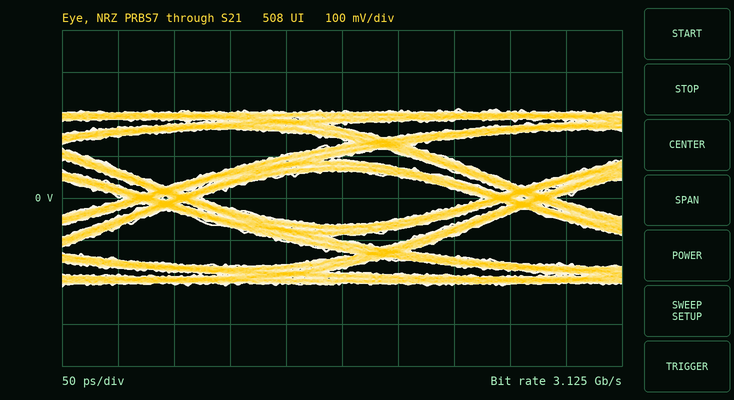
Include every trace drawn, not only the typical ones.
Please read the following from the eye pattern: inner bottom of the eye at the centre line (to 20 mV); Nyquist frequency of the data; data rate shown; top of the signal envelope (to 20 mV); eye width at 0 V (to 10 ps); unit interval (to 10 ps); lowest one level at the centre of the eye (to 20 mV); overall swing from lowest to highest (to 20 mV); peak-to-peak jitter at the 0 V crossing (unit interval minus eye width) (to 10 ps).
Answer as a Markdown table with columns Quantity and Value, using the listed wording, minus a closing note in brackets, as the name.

| Quantity | Value |
|---|---|
| inner bottom of the eye at the centre line | -60 mV |
| Nyquist frequency of the data | 1.5625 GHz |
| data rate shown | 3.125 Gb/s |
| top of the signal envelope | 220 mV |
| eye width at 0 V | 250 ps |
| unit interval | 320 ps |
| lowest one level at the centre of the eye | 60 mV |
| overall swing from lowest to highest | 420 mV |
| peak-to-peak jitter at the 0 V crossing (unit interval minus eye width) | 70 ps |
